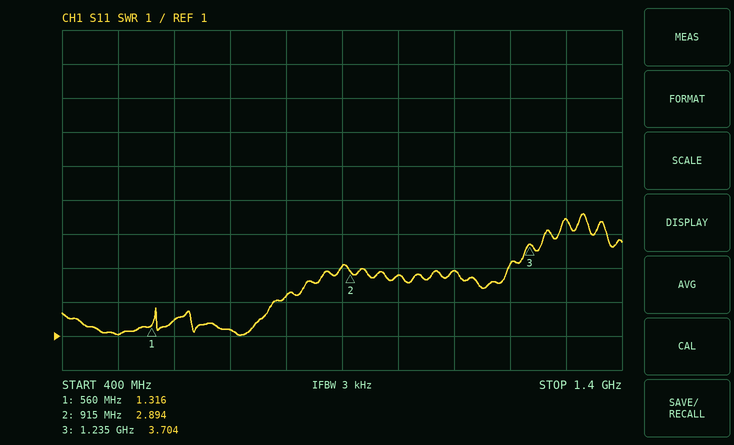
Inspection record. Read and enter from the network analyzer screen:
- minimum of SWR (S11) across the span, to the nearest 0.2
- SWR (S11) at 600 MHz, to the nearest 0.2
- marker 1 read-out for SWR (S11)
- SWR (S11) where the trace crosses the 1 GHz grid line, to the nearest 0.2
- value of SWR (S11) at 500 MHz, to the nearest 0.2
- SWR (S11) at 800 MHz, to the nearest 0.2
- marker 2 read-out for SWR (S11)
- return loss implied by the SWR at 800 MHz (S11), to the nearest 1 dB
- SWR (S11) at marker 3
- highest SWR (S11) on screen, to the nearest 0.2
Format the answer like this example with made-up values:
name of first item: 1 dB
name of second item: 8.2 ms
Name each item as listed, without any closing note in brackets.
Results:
minimum of SWR (S11) across the span, to the nearest 0.2: 1.0
SWR (S11) at 600 MHz, to the nearest 0.2: 1.4
marker 1 read-out for SWR: 1.316
SWR (S11) where the trace crosses the 1 GHz grid line, to the nearest 0.2: 2.8
value of SWR (S11) at 500 MHz, to the nearest 0.2: 1.0
SWR (S11) at 800 MHz, to the nearest 0.2: 2.2
marker 2 read-out for SWR: 2.894
return loss implied by the SWR at 800 MHz (S11), to the nearest 1 dB: 9 dB
SWR (S11) at marker 3: 3.704
highest SWR (S11) on screen, to the nearest 0.2: 4.6
